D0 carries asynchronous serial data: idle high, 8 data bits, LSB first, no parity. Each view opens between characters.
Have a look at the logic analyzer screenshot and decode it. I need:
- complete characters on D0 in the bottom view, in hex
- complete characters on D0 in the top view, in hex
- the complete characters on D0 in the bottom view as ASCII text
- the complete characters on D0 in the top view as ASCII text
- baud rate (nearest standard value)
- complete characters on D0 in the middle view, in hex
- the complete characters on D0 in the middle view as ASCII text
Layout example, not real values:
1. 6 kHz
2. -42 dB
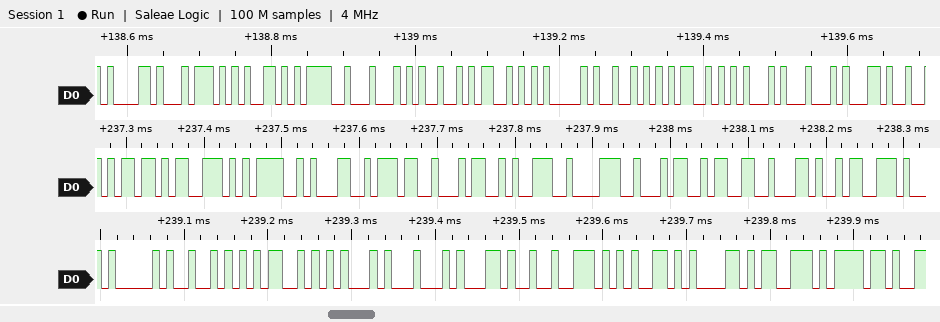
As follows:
1. 41, 52, 4D, 45, 44, 2C, 72, 65, 61, 73, 6F
2. 61, 74, 65, 3D, 44, 49, 53, 41, 52, 4D, 45, 44, 2C
3. "ARMED,reaso"
4. "ate=DISARMED,"
5. 115200 baud
6. 6D, 73, 3D, 31, 37, 34, 39, 38, 34, 33, 2C, 73
7. "ms=1749843,s"
